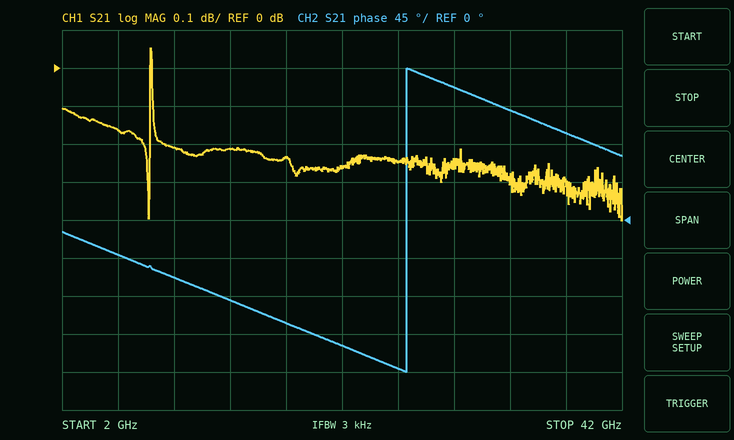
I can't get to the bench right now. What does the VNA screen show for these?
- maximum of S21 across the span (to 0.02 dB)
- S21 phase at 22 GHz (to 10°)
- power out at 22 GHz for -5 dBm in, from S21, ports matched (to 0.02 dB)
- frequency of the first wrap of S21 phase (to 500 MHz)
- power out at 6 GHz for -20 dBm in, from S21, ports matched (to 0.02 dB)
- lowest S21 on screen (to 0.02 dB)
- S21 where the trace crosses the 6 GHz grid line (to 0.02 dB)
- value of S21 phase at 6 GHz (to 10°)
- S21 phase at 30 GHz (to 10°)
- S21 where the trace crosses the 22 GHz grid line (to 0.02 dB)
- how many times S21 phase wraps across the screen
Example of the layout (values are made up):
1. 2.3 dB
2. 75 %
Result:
1. 0.06 dB
2. -150°
3. -5.26 dBm
4. 26.5 GHz
5. -20.16 dBm
6. -0.40 dB
7. -0.16 dB
8. -40°
9. 160°
10. -0.26 dB
11. 1
